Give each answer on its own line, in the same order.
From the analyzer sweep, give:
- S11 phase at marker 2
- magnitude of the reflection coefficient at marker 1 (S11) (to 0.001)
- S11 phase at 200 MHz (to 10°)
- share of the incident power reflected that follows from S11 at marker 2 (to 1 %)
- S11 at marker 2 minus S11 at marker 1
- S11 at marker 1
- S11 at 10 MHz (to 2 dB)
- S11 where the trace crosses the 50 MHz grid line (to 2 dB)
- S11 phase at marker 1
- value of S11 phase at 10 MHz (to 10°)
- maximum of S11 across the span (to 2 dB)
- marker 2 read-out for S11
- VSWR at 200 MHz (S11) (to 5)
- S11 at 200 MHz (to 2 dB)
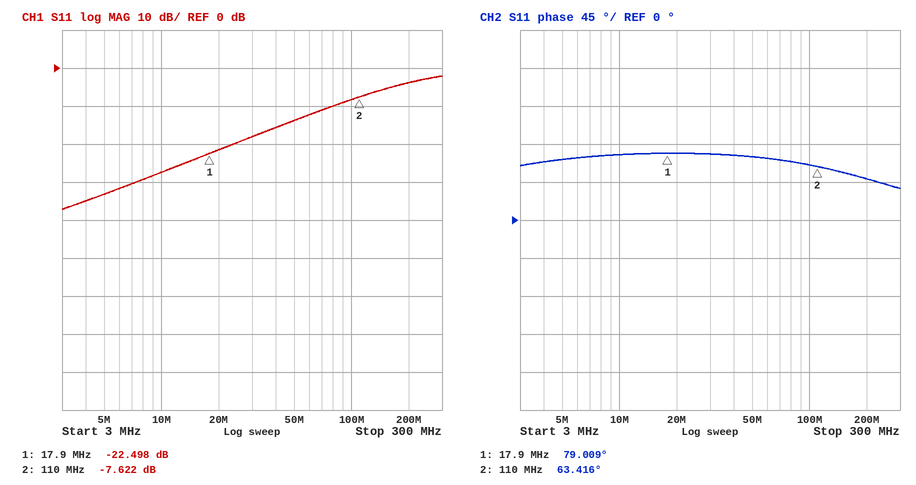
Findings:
63.416°
0.075
50°
17 %
14.876 dB
-22.498 dB
-28 dB
-14 dB
79.009°
80°
-2 dB
-7.622 dB
5
-4 dB
